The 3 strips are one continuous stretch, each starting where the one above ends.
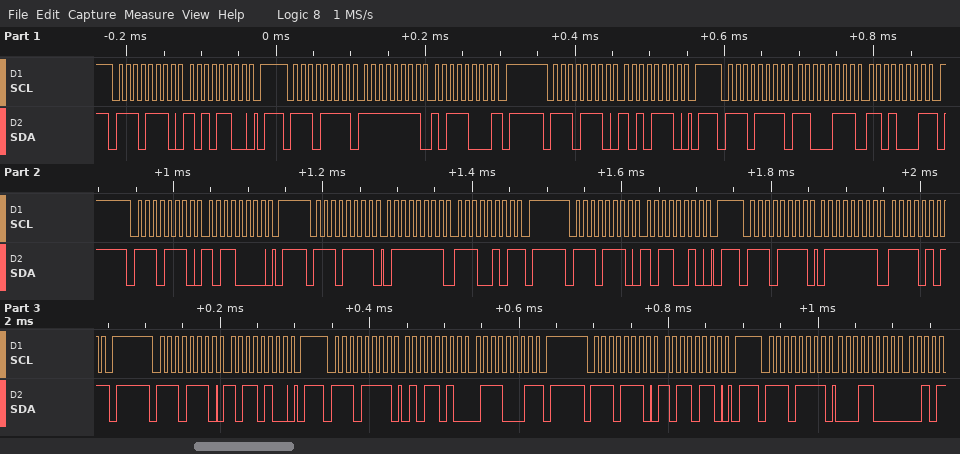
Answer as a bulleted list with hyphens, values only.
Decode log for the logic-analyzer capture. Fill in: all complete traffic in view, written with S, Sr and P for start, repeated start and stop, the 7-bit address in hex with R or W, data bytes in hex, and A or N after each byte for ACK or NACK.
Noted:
- S 77W A AC A P S 77R A FF A B8 N P S 77W A AE A P S 77R A C7 A D1 N P S 77W A B0 A P S 77R A 7F A E5 N P S 77W A B2 A P S 77R A 7F A F5 N P S 77W A B4 A P S 77R A 5A A 71 N P S 77W A B6 A P S 77R A 18 A
